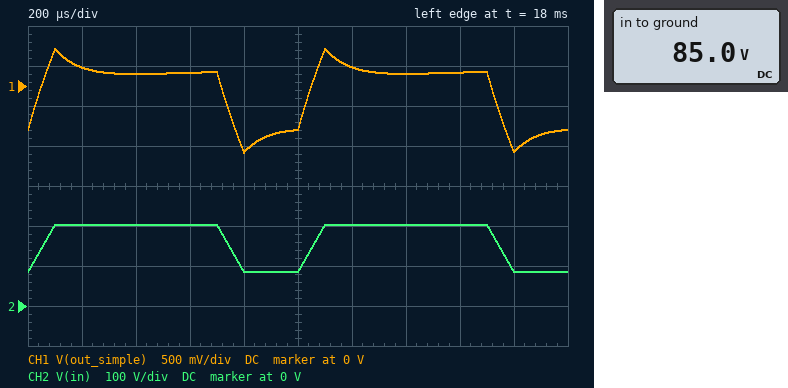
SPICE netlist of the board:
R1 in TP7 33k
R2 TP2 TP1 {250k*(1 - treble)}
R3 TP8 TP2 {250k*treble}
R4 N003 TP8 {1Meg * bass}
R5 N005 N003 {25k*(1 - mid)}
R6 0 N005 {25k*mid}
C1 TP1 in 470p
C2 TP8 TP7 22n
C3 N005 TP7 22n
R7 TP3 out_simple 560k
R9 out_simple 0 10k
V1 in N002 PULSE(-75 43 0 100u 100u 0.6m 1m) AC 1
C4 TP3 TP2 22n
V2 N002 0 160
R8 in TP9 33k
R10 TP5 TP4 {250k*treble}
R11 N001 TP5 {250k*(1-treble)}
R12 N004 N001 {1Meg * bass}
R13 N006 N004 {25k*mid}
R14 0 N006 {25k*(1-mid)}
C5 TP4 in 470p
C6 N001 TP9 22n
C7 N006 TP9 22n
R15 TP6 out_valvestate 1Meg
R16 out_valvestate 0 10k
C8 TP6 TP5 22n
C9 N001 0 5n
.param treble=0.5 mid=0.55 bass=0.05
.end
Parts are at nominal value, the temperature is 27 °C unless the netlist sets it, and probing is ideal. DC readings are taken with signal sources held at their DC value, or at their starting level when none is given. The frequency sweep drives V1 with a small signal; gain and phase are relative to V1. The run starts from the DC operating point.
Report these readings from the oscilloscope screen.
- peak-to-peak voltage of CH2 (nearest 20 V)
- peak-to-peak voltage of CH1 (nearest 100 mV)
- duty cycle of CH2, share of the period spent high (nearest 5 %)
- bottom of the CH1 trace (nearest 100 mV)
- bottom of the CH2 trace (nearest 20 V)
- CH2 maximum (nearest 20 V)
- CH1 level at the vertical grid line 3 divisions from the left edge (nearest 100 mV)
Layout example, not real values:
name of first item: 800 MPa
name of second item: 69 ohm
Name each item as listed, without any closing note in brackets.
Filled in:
peak-to-peak voltage of CH2: 120 V
peak-to-peak voltage of CH1: 1.3 V
duty cycle of CH2, share of the period spent high: 70 %
bottom of the CH1 trace: -800 mV
bottom of the CH2 trace: 80 V
CH2 maximum: 200 V
CH1 level at the vertical grid line 3 divisions from the left edge: 200 mV
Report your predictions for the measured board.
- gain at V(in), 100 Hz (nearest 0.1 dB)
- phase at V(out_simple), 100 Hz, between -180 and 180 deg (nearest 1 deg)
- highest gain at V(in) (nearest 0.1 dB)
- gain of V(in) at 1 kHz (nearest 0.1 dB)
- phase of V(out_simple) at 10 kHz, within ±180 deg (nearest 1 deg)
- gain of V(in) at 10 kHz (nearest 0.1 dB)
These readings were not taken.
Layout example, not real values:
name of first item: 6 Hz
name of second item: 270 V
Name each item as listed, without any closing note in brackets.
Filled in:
gain at V(in), 100 Hz: 0 dB
phase at V(out_simple), 100 Hz, between -180 and 180 deg: 29 deg
highest gain at V(in): 0 dB
gain of V(in) at 1 kHz: 0 dB
phase of V(out_simple) at 10 kHz, within ±180 deg: 4 deg
gain of V(in) at 10 kHz: 0 dB
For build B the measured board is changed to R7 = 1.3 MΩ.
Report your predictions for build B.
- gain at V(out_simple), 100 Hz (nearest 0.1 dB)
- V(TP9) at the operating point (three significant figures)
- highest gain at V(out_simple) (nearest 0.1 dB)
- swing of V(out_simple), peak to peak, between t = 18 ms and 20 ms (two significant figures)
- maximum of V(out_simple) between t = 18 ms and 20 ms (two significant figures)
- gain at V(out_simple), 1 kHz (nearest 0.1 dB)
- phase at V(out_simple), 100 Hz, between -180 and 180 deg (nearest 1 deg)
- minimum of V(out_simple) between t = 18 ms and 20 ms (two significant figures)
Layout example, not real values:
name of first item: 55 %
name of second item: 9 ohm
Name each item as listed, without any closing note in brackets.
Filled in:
gain at V(out_simple), 100 Hz: -48.0 dB
V(TP9) at the operating point: 85.0 V
highest gain at V(out_simple): -46.4 dB
swing of V(out_simple), peak to peak, between t = 18 ms and 20 ms: 590 mV
maximum of V(out_simple) between t = 18 ms and 20 ms: 210 mV
gain at V(out_simple), 1 kHz: -49.8 dB
phase at V(out_simple), 100 Hz, between -180 and 180 deg: 25 deg
minimum of V(out_simple) between t = 18 ms and 20 ms: -380 mV
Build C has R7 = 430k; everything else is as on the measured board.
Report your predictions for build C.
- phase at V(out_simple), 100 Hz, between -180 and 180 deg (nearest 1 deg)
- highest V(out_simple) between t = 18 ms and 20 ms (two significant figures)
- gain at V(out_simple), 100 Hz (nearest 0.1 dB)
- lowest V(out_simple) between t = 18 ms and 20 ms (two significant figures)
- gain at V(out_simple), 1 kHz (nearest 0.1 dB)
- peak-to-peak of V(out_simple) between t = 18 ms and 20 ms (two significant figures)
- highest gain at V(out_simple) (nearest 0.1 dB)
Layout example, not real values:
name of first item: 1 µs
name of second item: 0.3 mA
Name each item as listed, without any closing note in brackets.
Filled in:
phase at V(out_simple), 100 Hz, between -180 and 180 deg: 31 deg
highest V(out_simple) between t = 18 ms and 20 ms: 590 mV
gain at V(out_simple), 100 Hz: -40.4 dB
lowest V(out_simple) between t = 18 ms and 20 ms: -1.0 V
gain at V(out_simple), 1 kHz: -41.5 dB
peak-to-peak of V(out_simple) between t = 18 ms and 20 ms: 1.6 V
highest gain at V(out_simple): -37.7 dB
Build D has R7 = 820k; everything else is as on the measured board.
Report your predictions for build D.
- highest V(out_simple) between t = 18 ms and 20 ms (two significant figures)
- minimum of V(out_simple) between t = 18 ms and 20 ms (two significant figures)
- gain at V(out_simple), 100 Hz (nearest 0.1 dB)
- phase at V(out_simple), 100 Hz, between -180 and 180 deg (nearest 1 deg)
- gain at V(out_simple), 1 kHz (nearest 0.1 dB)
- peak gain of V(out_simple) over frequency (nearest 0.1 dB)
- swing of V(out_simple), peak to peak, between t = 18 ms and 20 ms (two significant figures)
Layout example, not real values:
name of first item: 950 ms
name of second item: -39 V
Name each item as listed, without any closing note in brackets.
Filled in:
highest V(out_simple) between t = 18 ms and 20 ms: 320 mV
minimum of V(out_simple) between t = 18 ms and 20 ms: -590 mV
gain at V(out_simple), 100 Hz: -44.6 dB
phase at V(out_simple), 100 Hz, between -180 and 180 deg: 27 deg
gain at V(out_simple), 1 kHz: -46.2 dB
peak gain of V(out_simple) over frequency: -42.6 dB
swing of V(out_simple), peak to peak, between t = 18 ms and 20 ms: 910 mV
